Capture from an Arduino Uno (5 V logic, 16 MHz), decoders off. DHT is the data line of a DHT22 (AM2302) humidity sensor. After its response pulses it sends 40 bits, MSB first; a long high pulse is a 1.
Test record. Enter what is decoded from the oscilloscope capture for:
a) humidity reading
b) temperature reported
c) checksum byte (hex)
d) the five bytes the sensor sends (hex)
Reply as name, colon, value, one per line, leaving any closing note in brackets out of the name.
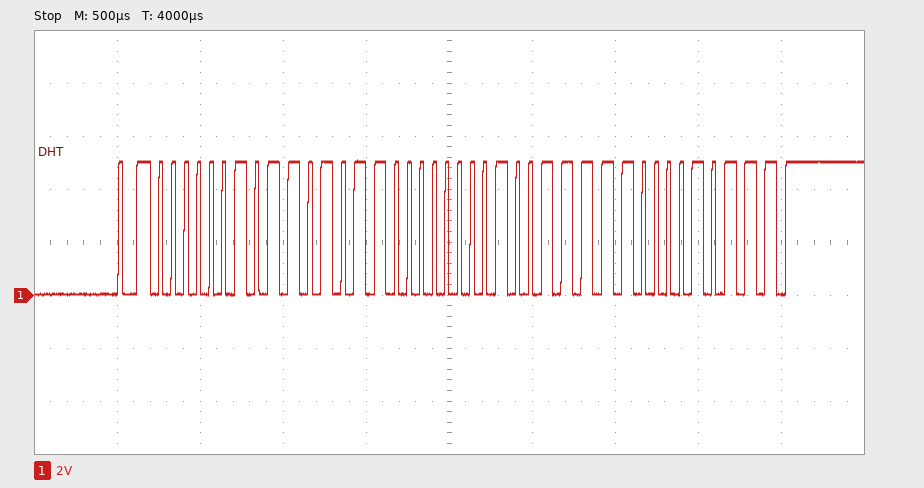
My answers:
humidity reading: 72.6 %
temperature reported: 31.8 °C
checksum byte: 0x17
the five bytes the sensor sends: 02 D6 01 3E 17
